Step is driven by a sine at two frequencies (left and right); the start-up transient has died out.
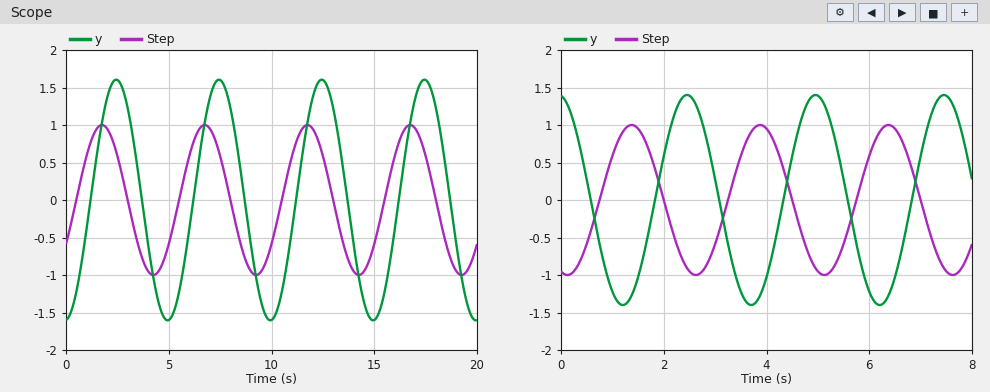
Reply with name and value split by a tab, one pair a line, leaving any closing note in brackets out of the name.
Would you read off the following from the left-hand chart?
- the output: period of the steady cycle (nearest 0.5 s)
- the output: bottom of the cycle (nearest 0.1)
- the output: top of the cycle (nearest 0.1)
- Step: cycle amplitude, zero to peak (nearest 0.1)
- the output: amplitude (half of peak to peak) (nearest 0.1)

the output: period of the steady cycle	5.0 s
the output: bottom of the cycle	-1.6
the output: top of the cycle	1.6
Step: cycle amplitude, zero to peak	1.0
the output: amplitude (half of peak to peak)	1.6
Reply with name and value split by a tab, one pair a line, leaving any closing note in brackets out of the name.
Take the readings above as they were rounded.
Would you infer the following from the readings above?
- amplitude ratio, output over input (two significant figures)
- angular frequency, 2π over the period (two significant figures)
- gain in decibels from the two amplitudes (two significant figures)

amplitude ratio, output over input	1.6
angular frequency, 2π over the period	1.3 rad/s
gain in decibels from the two amplitudes	4.1 dB
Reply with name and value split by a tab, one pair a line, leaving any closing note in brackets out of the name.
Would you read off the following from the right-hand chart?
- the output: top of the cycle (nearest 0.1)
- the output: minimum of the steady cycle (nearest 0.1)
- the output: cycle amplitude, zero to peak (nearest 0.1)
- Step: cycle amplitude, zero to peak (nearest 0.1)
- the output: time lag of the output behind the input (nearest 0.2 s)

the output: top of the cycle	1.4
the output: minimum of the steady cycle	-1.4
the output: cycle amplitude, zero to peak	1.4
Step: cycle amplitude, zero to peak	1.0
the output: time lag of the output behind the input	1.0 s
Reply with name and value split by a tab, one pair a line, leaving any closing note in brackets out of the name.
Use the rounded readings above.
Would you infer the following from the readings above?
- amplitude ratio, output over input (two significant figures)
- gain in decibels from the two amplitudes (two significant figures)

amplitude ratio, output over input	1.4
gain in decibels from the two amplitudes	2.9 dB
